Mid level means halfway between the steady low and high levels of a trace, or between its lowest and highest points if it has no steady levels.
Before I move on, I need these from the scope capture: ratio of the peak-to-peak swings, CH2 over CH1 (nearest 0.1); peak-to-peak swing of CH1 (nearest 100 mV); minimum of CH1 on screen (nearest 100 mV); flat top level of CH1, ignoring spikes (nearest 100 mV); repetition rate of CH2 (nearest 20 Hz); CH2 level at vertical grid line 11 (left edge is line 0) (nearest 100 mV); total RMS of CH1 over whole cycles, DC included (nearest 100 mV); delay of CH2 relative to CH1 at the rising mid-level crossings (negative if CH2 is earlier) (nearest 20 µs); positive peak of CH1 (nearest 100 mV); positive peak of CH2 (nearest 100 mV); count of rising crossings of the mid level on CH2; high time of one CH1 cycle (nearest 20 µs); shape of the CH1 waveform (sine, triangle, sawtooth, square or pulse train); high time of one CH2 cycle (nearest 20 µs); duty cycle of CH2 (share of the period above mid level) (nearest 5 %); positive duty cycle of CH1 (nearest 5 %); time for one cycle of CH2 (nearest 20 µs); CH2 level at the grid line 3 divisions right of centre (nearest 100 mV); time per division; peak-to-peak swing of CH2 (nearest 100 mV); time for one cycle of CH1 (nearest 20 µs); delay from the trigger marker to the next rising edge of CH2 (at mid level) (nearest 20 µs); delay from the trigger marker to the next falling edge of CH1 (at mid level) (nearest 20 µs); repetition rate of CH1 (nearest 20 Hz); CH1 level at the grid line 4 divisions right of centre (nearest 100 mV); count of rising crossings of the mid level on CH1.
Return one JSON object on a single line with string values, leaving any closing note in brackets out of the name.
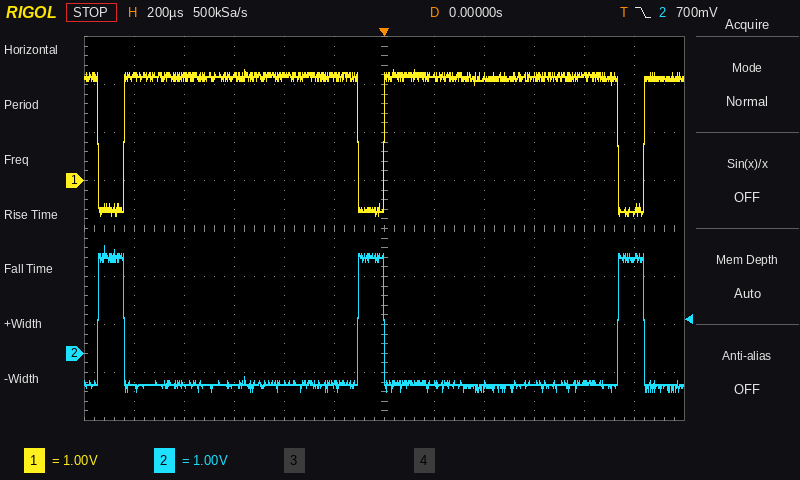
{"ratio of the peak-to-peak swings, CH2 over CH1": "1.0", "peak-to-peak swing of CH1": "3.0 V", "minimum of CH1 on screen": "-700 mV", "flat top level of CH1, ignoring spikes": "2.2 V", "repetition rate of CH2": "960 Hz", "CH2 level at vertical grid line 11 (left edge is line 0)": "2.0 V", "total RMS of CH1 over whole cycles, DC included": "2.1 V", "delay of CH2 relative to CH1 at the rising mid-level crossings (negative if CH2 is earlier)": "-100 µs", "positive peak of CH1": "2.3 V", "positive peak of CH2": "2.2 V", "count of rising crossings of the mid level on CH2": "3", "high time of one CH1 cycle": "940 µs", "shape of the CH1 waveform": "pulse train", "high time of one CH2 cycle": "100 µs", "duty cycle of CH2 (share of the period above mid level)": "10 %", "positive duty cycle of CH1": "90 %", "time for one cycle of CH2": "1.04 ms", "CH2 level at the grid line 3 divisions right of centre": "-600 mV", "time per division": "200 µs", "peak-to-peak swing of CH2": "3.0 V", "time for one cycle of CH1": "1.04 ms", "delay from the trigger marker to the next rising edge of CH2 (at mid level)": "940 µs", "delay from the trigger marker to the next falling edge of CH1 (at mid level)": "940 µs", "repetition rate of CH1": "960 Hz", "CH1 level at the grid line 4 divisions right of centre": "2.2 V", "count of rising crossings of the mid level on CH1": "3"}
